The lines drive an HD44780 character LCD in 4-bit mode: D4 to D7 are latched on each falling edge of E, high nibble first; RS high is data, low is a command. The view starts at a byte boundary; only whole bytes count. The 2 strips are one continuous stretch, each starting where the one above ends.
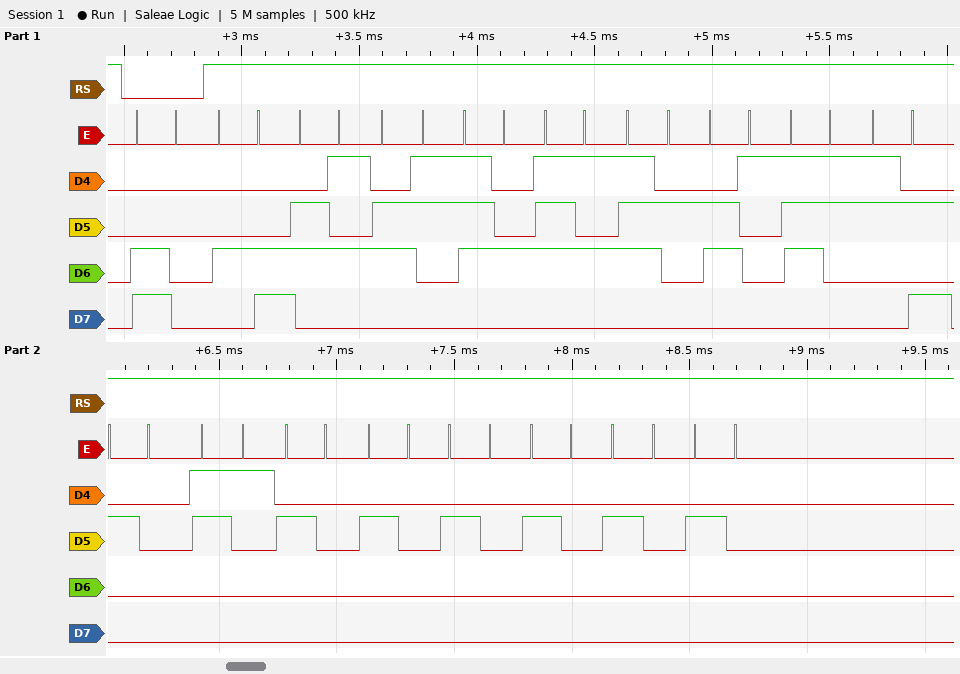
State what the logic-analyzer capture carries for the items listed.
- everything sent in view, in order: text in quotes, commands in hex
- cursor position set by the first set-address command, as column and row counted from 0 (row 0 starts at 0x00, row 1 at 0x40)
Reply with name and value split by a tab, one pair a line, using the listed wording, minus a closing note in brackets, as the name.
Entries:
everything sent in view, in order: text in quotes, commands in hex	0xC0 "Lecturas: 1      "
cursor position set by the first set-address command, as column and row counted from 0	column 0, row 1
